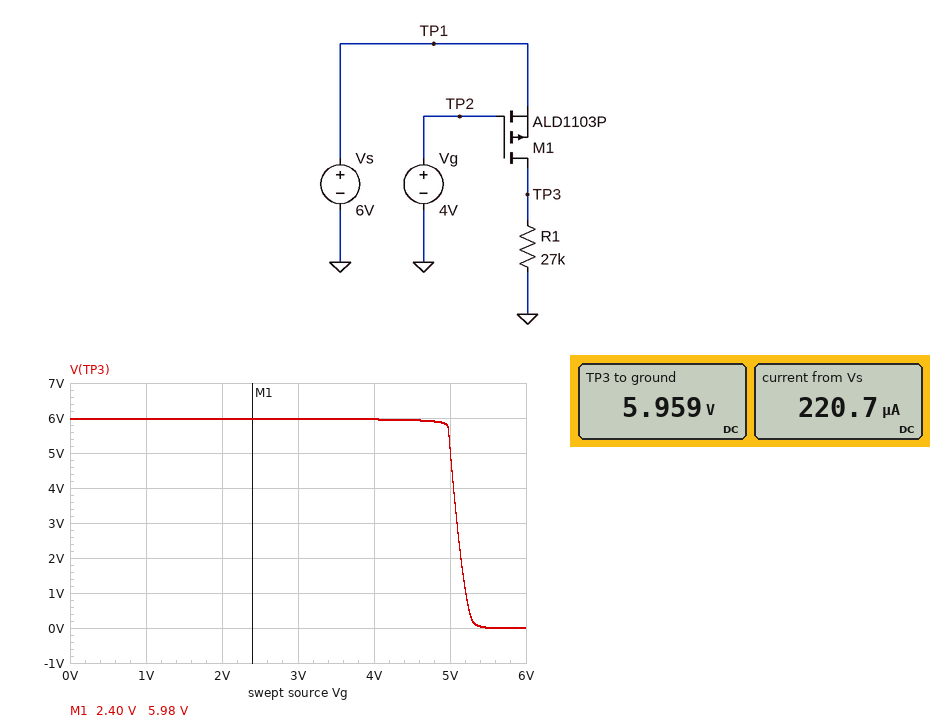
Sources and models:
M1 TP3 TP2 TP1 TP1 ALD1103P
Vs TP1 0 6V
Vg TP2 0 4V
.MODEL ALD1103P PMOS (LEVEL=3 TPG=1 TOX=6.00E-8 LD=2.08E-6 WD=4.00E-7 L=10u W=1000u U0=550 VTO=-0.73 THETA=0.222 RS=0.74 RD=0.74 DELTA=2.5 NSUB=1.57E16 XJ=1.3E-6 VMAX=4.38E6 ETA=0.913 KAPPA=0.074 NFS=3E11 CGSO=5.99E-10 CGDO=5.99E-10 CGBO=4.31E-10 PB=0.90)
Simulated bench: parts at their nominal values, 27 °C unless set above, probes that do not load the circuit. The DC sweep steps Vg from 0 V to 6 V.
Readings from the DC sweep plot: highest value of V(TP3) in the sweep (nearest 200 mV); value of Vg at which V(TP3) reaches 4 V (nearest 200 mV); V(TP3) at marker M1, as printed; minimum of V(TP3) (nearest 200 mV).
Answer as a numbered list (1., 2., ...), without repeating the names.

1. 6.0 V
2. 5.0 V
3. 5.98 V
4. 0 V
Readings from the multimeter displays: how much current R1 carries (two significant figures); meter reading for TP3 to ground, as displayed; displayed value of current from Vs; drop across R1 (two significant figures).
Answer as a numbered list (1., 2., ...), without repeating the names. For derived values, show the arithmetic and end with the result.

1. (5.959 V) / 27 kΩ = 220 µA
2. 5.959 V
3. 220.7 µA
4. 5.959 V = 6.0 V
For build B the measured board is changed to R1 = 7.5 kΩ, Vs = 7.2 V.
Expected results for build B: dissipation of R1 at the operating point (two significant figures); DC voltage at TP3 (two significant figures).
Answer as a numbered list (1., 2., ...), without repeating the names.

1. 6.7 mW
2. 7.1 V
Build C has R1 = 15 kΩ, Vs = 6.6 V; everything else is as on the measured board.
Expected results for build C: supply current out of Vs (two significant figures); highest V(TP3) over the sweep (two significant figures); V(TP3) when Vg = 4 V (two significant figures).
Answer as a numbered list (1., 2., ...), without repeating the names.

1. 440 µA
2. 6.6 V
3. 6.5 V
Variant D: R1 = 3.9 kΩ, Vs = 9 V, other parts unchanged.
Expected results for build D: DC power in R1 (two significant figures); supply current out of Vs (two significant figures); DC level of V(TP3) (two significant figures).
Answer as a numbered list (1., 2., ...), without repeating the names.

1. 20 mW
2. 2.3 mA
3. 8.8 V
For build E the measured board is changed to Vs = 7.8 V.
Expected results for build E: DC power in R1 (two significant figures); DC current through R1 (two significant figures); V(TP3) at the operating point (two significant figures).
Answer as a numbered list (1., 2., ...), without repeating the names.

1. 2.2 mW
2. 290 µA
3. 7.8 V
